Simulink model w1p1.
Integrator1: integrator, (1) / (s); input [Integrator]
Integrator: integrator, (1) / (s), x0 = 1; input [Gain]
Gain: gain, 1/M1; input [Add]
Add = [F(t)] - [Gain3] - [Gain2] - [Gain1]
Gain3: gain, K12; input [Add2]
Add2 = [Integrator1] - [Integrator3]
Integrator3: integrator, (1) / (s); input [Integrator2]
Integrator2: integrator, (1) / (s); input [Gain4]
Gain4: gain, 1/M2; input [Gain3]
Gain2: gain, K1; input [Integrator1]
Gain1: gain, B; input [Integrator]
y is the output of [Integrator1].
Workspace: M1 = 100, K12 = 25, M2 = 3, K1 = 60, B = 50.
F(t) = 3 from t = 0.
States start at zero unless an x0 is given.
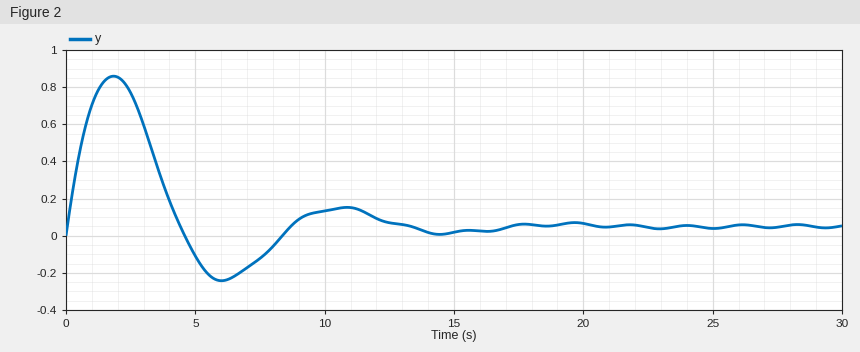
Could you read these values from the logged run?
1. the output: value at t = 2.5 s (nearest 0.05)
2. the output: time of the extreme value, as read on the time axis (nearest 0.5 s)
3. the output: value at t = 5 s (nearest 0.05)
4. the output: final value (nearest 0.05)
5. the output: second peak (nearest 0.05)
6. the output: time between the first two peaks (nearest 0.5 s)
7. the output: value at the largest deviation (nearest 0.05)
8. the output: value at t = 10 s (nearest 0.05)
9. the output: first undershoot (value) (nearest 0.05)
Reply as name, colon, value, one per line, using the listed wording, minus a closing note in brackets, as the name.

the output: value at t = 2.5 s: 0.75
the output: time of the extreme value, as read on the time axis: 2.0 s
the output: value at t = 5 s: -0.10
the output: final value: 0.05
the output: second peak: 0.15
the output: time between the first two peaks: 9.0 s
the output: value at the largest deviation: 0.85
the output: value at t = 10 s: 0.15
the output: first undershoot (value): -0.25
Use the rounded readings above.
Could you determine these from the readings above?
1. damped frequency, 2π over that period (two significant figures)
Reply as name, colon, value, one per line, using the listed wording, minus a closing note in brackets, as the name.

damped frequency, 2π over that period: 0.70 rad/s
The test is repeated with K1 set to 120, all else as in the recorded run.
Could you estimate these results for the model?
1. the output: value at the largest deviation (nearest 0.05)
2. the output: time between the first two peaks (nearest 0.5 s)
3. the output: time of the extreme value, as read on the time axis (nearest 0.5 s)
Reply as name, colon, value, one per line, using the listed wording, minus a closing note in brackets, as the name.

the output: value at the largest deviation: 0.65
the output: time between the first two peaks: 6.0 s
the output: time of the extreme value, as read on the time axis: 1.5 s
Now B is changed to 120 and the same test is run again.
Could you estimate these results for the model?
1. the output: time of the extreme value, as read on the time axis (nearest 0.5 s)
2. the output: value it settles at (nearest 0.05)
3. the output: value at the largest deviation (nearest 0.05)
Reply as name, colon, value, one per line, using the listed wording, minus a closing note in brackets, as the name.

the output: time of the extreme value, as read on the time axis: 1.5 s
the output: value it settles at: 0.05
the output: value at the largest deviation: 0.55
